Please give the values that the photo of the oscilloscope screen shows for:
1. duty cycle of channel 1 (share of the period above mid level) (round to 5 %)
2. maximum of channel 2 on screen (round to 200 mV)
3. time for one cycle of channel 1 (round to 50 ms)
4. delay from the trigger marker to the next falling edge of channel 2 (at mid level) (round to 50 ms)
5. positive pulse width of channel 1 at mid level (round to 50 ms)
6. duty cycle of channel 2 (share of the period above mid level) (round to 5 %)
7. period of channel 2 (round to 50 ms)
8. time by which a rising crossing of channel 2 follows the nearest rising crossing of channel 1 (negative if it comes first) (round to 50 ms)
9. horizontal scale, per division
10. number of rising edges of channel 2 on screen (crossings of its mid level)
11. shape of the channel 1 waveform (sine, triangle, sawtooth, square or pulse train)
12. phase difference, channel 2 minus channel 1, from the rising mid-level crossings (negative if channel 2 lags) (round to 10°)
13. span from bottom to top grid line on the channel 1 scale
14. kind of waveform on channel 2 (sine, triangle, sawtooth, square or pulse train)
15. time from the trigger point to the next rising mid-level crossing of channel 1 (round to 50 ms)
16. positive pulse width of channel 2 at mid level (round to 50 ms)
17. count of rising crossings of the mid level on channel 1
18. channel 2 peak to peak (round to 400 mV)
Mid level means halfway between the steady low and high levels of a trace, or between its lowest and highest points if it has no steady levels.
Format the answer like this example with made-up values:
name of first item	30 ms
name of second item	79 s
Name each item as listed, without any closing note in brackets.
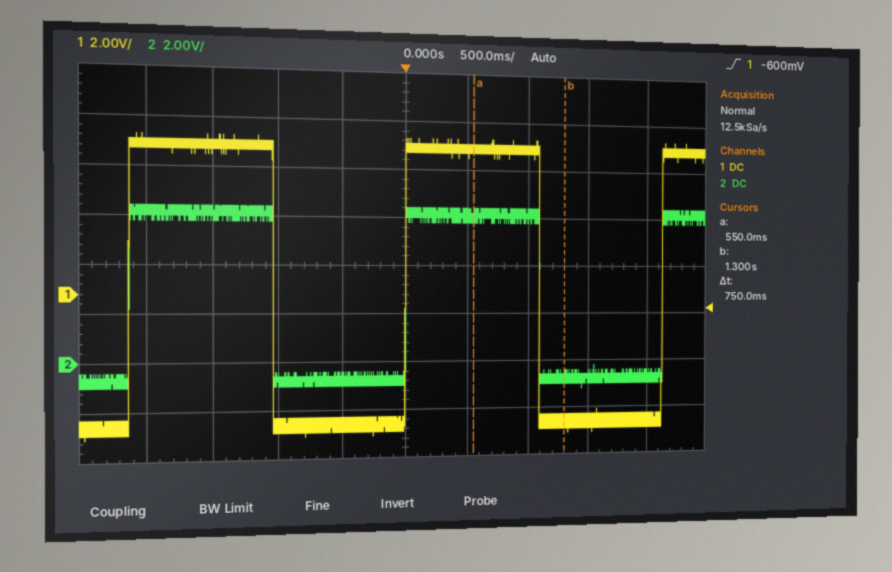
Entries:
duty cycle of channel 1 (share of the period above mid level)	50 %
maximum of channel 2 on screen	6.4 V
time for one cycle of channel 1	2.15 s
delay from the trigger marker to the next falling edge of channel 2 (at mid level)	1.10 s
positive pulse width of channel 1 at mid level	1.10 s
duty cycle of channel 2 (share of the period above mid level)	50 %
period of channel 2	2.15 s
time by which a rising crossing of channel 2 follows the nearest rising crossing of channel 1 (negative if it comes first)	0 ms
horizontal scale, per division	500 ms
number of rising edges of channel 2 on screen	3
shape of the channel 1 waveform	square
phase difference, channel 2 minus channel 1, from the rising mid-level crossings (negative if channel 2 lags)	0°
span from bottom to top grid line on the channel 1 scale	16 V
kind of waveform on channel 2	square
time from the trigger point to the next rising mid-level crossing of channel 1	2.15 s
positive pulse width of channel 2 at mid level	1.10 s
count of rising crossings of the mid level on channel 1	3
channel 2 peak to peak	7.6 V
